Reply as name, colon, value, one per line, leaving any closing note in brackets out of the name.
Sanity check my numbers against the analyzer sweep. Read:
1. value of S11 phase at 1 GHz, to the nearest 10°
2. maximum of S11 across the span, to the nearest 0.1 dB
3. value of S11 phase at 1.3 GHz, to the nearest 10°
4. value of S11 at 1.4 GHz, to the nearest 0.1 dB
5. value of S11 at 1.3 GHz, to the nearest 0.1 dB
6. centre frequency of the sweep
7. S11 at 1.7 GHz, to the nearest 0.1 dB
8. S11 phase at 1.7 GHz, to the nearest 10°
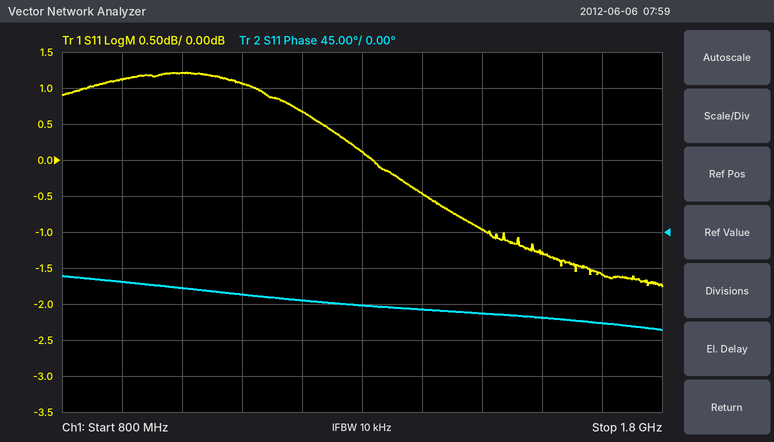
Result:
value of S11 phase at 1 GHz, to the nearest 10°: -70°
maximum of S11 across the span, to the nearest 0.1 dB: 1.2 dB
value of S11 phase at 1.3 GHz, to the nearest 10°: -90°
value of S11 at 1.4 GHz, to the nearest 0.1 dB: -0.5 dB
value of S11 at 1.3 GHz, to the nearest 0.1 dB: 0.1 dB
centre frequency of the sweep: 1.3 GHz
S11 at 1.7 GHz, to the nearest 0.1 dB: -1.6 dB
S11 phase at 1.7 GHz, to the nearest 10°: -110°
